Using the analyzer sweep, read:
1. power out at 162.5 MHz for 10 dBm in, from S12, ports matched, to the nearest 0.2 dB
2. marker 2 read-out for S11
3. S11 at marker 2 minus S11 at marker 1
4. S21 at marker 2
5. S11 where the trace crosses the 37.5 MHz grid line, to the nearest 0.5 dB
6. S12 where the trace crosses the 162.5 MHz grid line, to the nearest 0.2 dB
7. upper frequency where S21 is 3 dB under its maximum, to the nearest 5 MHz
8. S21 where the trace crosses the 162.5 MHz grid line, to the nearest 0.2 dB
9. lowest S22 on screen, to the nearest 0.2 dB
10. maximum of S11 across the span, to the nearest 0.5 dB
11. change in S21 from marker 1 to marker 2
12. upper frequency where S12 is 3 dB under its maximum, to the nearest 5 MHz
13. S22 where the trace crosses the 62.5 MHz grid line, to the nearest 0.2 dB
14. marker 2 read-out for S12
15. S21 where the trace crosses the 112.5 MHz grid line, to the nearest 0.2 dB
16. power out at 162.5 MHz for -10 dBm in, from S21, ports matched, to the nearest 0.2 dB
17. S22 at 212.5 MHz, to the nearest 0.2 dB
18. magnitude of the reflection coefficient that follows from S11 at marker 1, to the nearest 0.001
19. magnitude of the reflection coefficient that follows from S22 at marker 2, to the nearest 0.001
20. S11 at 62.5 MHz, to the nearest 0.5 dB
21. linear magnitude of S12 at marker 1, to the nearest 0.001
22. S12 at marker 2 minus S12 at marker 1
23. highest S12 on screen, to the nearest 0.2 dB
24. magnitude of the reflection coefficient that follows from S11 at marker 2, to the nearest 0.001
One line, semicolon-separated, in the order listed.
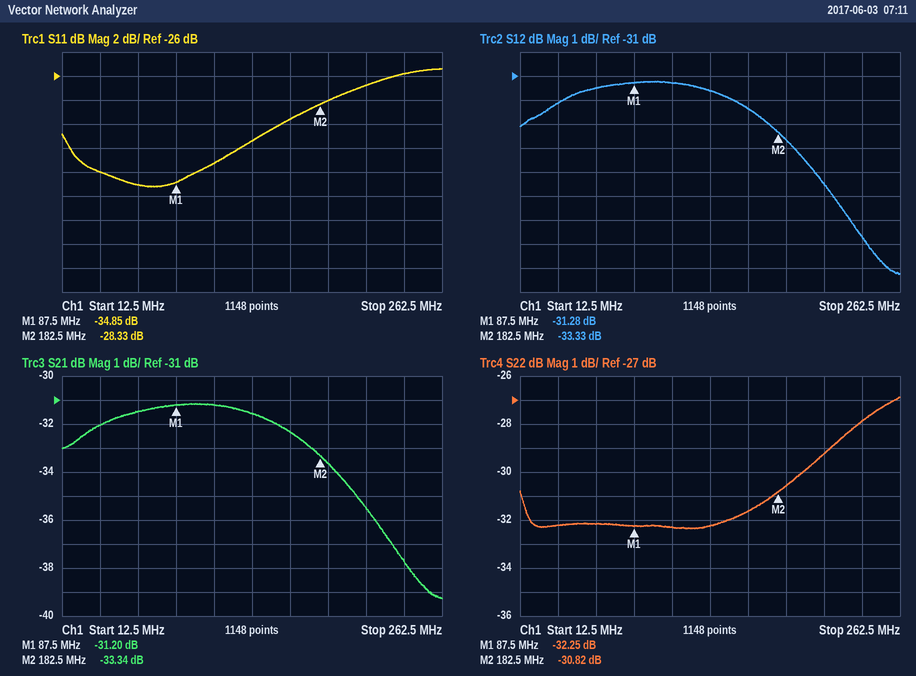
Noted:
-22.4 dBm; -28.33 dB; 6.52 dB; -33.34 dB; -34.0 dB; -32.4 dB; 195 MHz; -32.4 dB; -32.4 dB; -25.5 dB; -2.14 dB; 195 MHz; -32.2 dB; -33.33 dB; -31.2 dB; -42.4 dBm; -29.2 dB; 0.018; 0.029; -35.0 dB; 0.027; -2.05 dB; -31.2 dB; 0.038
